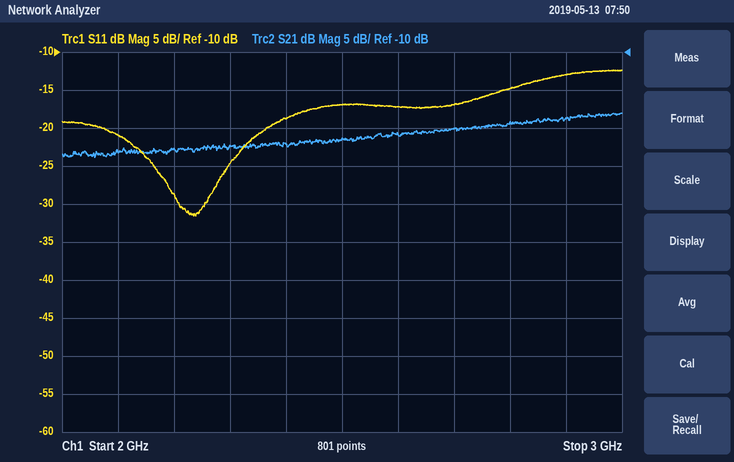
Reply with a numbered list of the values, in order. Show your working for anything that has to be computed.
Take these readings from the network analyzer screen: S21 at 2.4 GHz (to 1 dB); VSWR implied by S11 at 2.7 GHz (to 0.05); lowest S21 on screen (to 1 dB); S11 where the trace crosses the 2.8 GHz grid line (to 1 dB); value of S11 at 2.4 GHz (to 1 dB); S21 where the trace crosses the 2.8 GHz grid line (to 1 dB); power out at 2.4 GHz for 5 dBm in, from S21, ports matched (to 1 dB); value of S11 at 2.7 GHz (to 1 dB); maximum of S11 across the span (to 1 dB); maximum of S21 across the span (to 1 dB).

1. -22 dB
2. |Γ| = 10^(-17/20) = 0.1413; VSWR = (1 + 0.1413)/(1 − 0.1413) ≈ 1.33, so 1.35 to the nearest 0.05
3. -24 dB
4. -15 dB
5. -19 dB
6. -19 dB
7. 5 dBm + (-22 dB) = -17 dBm
8. -17 dB
9. -12 dB
10. -18 dB
